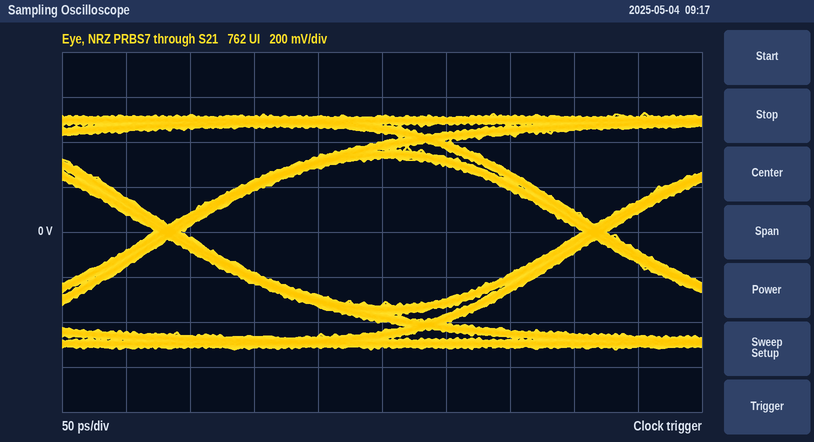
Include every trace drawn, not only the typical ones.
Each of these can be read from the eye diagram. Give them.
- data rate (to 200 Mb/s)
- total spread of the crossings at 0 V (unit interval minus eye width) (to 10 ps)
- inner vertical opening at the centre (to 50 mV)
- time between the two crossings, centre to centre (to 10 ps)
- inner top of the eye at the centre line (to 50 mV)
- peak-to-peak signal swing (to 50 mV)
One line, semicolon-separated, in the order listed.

3.0 Gb/s; 20 ps; 650 mV; 330 ps; 350 mV; 1.05 V
